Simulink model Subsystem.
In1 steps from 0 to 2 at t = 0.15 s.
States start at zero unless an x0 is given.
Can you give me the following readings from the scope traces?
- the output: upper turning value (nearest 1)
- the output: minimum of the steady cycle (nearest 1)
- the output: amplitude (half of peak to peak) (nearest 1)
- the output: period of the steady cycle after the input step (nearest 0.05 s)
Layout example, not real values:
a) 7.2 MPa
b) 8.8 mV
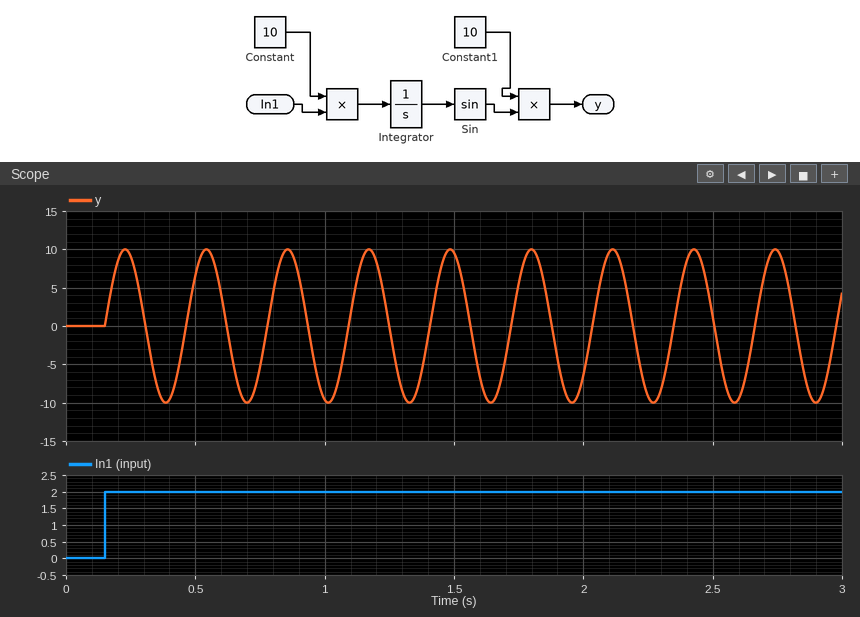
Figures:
a) 10
b) -10
c) 10
d) 0.30 s
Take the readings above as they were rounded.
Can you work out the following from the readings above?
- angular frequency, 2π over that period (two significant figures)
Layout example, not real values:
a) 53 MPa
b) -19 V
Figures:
a) 21 rad/s
